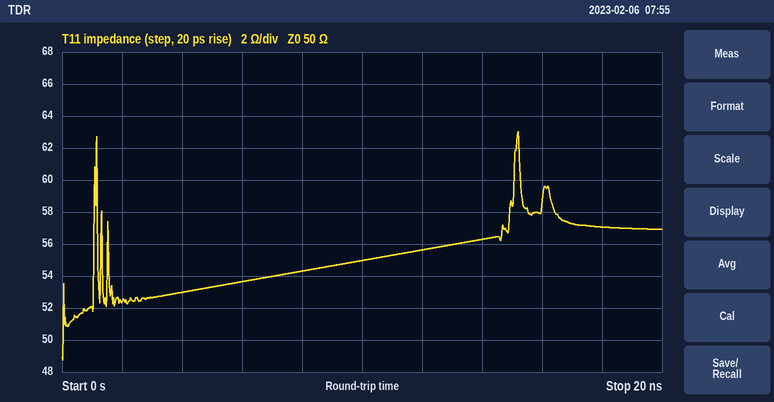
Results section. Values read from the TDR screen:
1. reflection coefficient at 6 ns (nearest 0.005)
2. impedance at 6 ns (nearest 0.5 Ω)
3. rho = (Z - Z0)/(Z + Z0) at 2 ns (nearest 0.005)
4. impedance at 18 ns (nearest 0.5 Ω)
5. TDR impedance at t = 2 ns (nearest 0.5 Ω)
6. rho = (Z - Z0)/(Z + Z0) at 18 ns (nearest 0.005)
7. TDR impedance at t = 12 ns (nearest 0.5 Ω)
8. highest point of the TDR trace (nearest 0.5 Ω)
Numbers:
+0.035
53.5 Ω
+0.025
57.0 Ω
52.5 Ω
+0.065
55.5 Ω
63.0 Ω
